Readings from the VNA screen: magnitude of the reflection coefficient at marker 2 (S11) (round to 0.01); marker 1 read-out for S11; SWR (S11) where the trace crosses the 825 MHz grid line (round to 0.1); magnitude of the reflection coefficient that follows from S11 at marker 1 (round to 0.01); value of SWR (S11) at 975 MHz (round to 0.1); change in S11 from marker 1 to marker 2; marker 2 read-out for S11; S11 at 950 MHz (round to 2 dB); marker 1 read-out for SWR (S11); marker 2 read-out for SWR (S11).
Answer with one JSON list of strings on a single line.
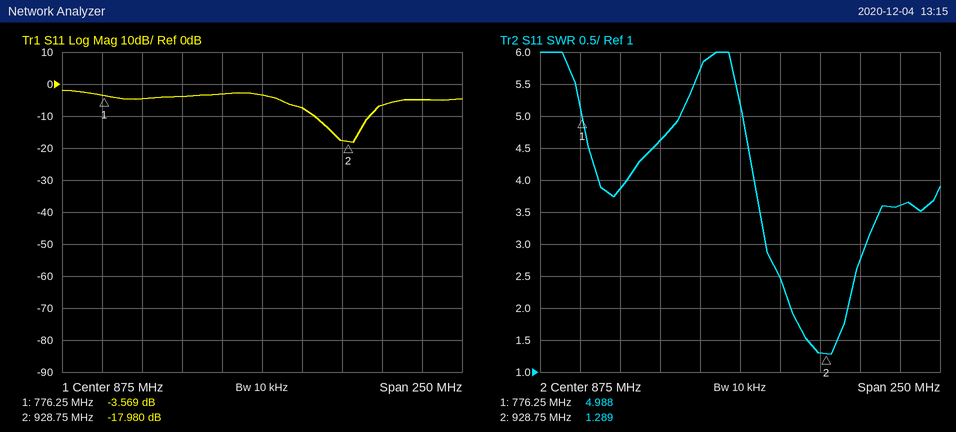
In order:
["0.13", "-3.569 dB", "4.6", "0.66", "3.6", "-14.411 dB", "-17.980 dB", "-6 dB", "4.988", "1.289"]
